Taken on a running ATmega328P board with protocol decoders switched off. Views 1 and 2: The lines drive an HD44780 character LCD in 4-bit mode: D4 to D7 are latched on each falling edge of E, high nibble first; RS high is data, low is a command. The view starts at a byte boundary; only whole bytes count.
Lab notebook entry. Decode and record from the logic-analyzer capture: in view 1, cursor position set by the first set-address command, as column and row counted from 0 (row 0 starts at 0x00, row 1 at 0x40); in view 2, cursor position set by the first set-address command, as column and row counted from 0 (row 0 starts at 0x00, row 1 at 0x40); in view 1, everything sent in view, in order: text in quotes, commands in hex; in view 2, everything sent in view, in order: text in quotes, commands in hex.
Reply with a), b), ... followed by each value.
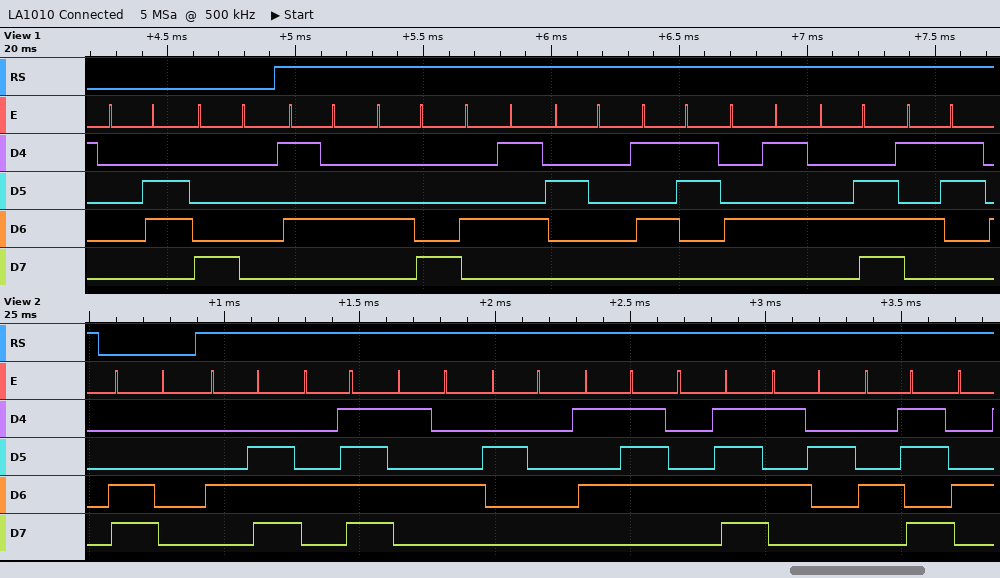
a) column 0, row 0
b) column 0, row 1
c) 0x06 0x80 "THE SENS"
d) 0xC0 "NOT WORK"
